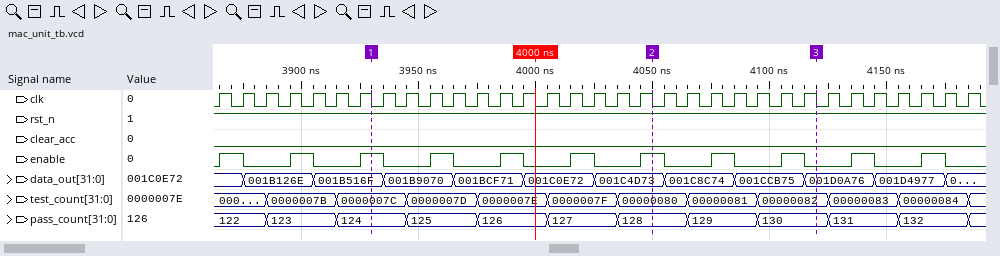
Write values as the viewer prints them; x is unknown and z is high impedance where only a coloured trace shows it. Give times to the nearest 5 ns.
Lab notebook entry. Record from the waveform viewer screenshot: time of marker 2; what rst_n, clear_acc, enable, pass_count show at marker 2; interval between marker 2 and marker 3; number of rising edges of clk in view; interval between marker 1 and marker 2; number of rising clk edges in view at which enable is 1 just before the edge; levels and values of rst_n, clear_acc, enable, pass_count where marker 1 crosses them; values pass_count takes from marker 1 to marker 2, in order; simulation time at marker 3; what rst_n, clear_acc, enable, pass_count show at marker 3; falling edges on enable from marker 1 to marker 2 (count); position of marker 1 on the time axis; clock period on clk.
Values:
4050 ns
rst_n=1, clear_acc=0, enable=1, pass_count=128
70 ns
33
120 ns
11
rst_n=1, clear_acc=0, enable=1, pass_count=124
124, 125, 126, 127, 128
4120 ns
rst_n=1, clear_acc=0, enable=0, pass_count=130
4
3930 ns
10 ns
